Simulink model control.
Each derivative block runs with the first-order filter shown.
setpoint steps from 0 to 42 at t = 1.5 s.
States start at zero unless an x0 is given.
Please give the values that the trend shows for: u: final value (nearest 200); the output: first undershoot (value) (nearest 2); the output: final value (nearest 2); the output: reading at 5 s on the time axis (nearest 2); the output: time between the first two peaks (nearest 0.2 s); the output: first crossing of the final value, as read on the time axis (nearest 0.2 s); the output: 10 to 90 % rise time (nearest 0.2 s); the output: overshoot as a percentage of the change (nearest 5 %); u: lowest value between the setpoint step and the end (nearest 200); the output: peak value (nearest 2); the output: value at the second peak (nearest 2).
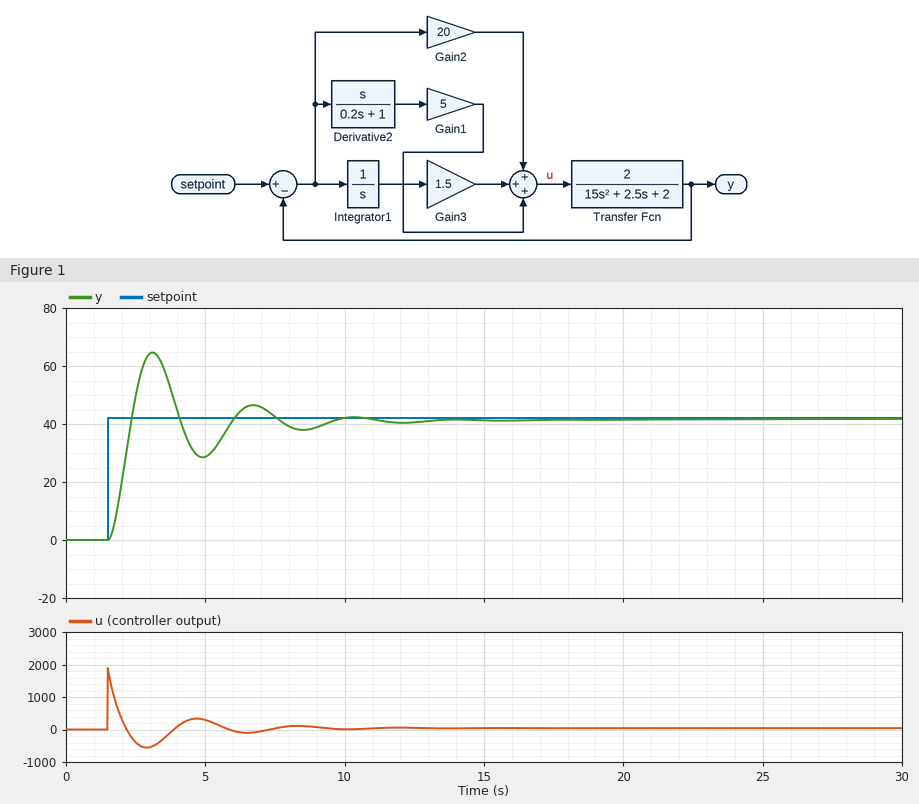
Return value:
0
28
42
28
3.6 s
2.4 s
0.6 s
55 %
-600
64
46
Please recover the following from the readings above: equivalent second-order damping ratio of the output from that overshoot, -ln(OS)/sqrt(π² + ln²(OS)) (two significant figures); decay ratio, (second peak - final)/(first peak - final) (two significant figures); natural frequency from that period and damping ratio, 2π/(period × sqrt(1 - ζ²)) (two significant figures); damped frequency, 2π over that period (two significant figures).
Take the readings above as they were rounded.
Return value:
0.19
0.18
1.8 rad/s
1.7 rad/s
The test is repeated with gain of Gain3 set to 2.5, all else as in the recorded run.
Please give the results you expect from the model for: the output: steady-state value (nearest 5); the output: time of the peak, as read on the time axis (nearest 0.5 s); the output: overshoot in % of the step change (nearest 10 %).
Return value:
40
3.0 s
60 %
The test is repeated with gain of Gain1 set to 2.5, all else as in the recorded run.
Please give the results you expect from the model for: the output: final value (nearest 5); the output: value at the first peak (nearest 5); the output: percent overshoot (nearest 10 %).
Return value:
40
70
70 %
